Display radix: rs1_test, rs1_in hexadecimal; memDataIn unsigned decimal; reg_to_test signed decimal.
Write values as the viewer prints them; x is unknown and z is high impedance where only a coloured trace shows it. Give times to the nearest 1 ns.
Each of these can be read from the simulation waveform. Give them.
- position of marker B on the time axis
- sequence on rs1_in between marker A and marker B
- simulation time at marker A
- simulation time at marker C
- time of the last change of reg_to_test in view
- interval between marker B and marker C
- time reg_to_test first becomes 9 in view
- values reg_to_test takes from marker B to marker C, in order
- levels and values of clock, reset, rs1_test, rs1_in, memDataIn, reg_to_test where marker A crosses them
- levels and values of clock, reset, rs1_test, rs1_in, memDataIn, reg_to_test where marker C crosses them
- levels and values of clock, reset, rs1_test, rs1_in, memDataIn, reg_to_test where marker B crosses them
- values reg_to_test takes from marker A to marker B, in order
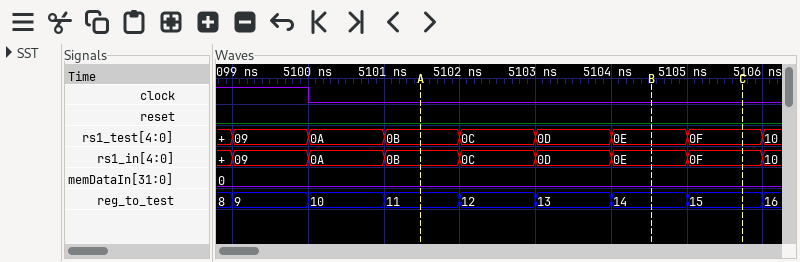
5105 ns
0B, 0C, 0D, 0E
5101 ns
5106 ns
5106 ns
1 ns
5099 ns
14, 15
clock=0, reset=0, rs1_test=0B, rs1_in=0B, memDataIn=0, reg_to_test=11
clock=0, reset=0, rs1_test=0F, rs1_in=0F, memDataIn=0, reg_to_test=15
clock=0, reset=0, rs1_test=0E, rs1_in=0E, memDataIn=0, reg_to_test=14
11, 12, 13, 14
